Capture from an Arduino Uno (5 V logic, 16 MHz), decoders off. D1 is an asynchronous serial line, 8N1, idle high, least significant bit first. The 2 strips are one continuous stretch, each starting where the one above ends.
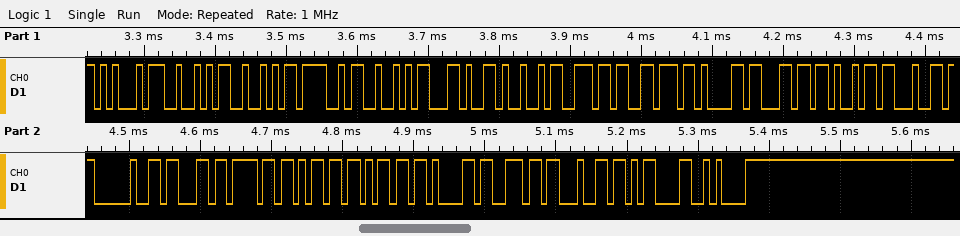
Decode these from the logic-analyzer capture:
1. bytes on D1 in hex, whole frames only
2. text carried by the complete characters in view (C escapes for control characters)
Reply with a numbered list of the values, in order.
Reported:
1. 45 52 52 4F 52 2C 49 6E 76 61 6C 69 64 20 63 6F 6D 6D 61 6E 64 0D 0A
2. "ERROR,Invalid command\r\n"
